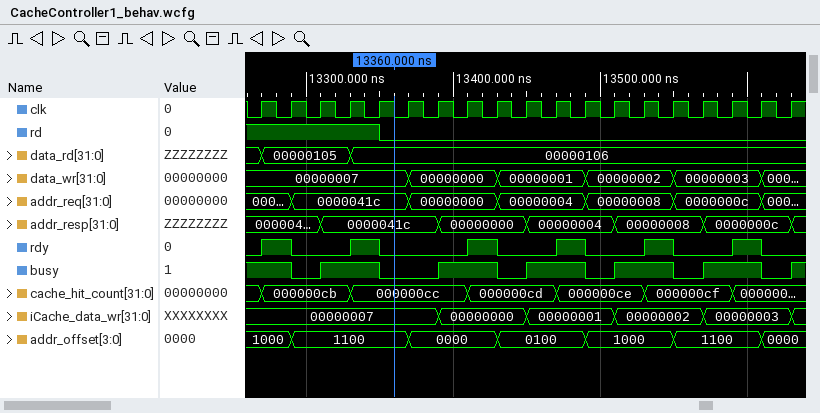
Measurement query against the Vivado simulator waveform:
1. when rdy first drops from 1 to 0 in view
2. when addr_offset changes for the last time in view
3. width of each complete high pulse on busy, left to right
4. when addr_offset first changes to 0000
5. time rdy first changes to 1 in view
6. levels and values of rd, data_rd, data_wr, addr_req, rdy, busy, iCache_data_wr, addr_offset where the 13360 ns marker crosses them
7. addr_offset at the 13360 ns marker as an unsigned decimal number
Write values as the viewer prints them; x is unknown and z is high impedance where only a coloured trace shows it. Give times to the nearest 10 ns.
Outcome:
13290 ns
13610 ns
40 ns, 40 ns, 40 ns, 40 ns, 40 ns
13370 ns
13270 ns
rd=0, data_rd=00000106, data_wr=00000007, addr_req=0000041c, rdy=0, busy=0, iCache_data_wr=00000007, addr_offset=1100
12
